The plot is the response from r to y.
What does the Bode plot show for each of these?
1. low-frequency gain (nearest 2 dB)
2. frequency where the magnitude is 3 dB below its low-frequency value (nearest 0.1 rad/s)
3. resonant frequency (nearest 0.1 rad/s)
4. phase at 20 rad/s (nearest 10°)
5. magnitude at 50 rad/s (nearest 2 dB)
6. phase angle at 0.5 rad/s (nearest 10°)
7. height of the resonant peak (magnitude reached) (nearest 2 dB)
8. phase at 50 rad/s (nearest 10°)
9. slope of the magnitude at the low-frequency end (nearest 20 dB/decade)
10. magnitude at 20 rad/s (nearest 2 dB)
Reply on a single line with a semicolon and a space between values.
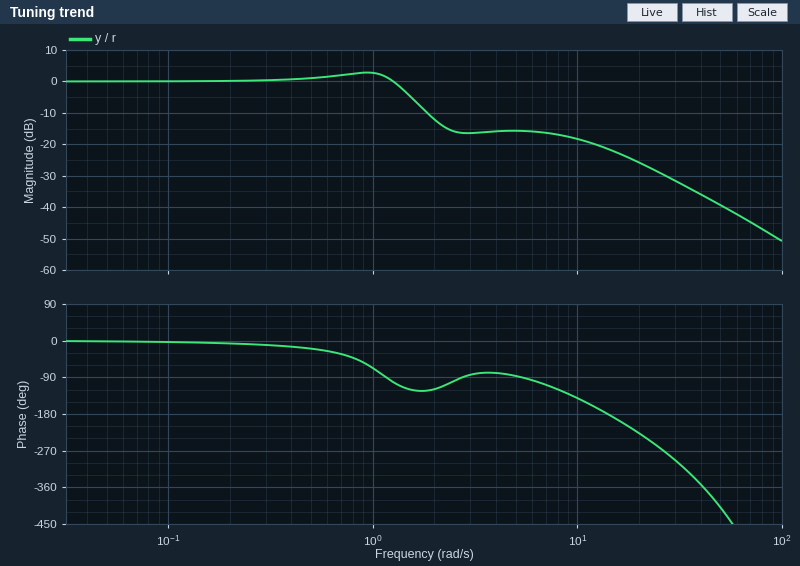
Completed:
0 dB; 1.4 rad/s; 0.9 rad/s; -230°; -40 dB; -20°; 2 dB; -410°; 0 dB/decade; -26 dB
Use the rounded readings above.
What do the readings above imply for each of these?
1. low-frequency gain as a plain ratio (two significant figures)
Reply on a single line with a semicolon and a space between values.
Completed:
1.0
